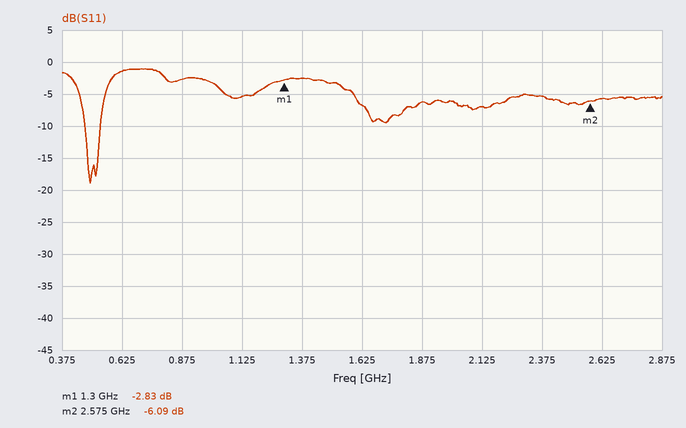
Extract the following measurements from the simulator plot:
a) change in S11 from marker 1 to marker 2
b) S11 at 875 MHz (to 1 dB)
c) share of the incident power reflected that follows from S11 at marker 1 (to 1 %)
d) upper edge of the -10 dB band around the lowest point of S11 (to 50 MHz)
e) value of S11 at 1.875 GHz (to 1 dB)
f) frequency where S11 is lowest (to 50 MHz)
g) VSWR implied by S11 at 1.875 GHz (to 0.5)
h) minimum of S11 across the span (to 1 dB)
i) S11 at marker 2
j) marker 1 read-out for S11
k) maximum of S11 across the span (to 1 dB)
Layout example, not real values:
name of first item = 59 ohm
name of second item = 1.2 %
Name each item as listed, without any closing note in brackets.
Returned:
change in S11 from marker 1 to marker 2 = -3.26 dB
S11 at 875 MHz = -3 dB
share of the incident power reflected that follows from S11 at marker 1 = 52 %
upper edge of the -10 dB band around the lowest point of S11 = 550 MHz
value of S11 at 1.875 GHz = -6 dB
frequency where S11 is lowest = 500 MHz
VSWR implied by S11 at 1.875 GHz = 3.0
minimum of S11 across the span = -19 dB
S11 at marker 2 = -6.09 dB
marker 1 read-out for S11 = -2.83 dB
maximum of S11 across the span = -1 dB
